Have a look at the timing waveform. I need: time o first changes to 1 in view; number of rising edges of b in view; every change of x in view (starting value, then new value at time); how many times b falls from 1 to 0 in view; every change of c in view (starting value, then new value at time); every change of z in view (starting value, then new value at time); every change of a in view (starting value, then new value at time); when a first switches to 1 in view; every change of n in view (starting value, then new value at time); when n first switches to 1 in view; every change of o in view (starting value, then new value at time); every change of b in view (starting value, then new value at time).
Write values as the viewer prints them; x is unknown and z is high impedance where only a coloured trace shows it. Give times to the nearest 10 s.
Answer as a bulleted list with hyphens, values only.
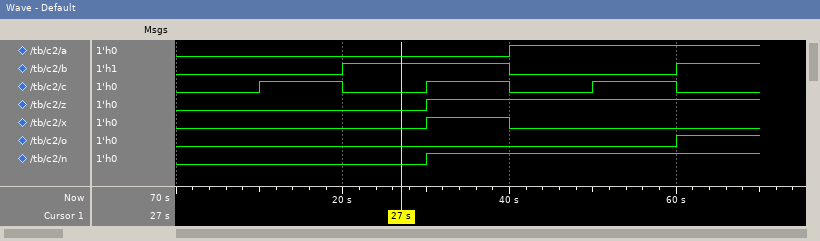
- 60 s
- 2
- 0, 1 at 30 s, 0 at 40 s
- 1
- 0, 1 at 10 s, 0 at 20 s, 1 at 30 s, 0 at 40 s, 1 at 50 s, 0 at 60 s
- 0, 1 at 30 s
- 0, 1 at 40 s
- 40 s
- 0, 1 at 30 s
- 30 s
- 0, 1 at 60 s
- 0, 1 at 20 s, 0 at 40 s, 1 at 60 s
